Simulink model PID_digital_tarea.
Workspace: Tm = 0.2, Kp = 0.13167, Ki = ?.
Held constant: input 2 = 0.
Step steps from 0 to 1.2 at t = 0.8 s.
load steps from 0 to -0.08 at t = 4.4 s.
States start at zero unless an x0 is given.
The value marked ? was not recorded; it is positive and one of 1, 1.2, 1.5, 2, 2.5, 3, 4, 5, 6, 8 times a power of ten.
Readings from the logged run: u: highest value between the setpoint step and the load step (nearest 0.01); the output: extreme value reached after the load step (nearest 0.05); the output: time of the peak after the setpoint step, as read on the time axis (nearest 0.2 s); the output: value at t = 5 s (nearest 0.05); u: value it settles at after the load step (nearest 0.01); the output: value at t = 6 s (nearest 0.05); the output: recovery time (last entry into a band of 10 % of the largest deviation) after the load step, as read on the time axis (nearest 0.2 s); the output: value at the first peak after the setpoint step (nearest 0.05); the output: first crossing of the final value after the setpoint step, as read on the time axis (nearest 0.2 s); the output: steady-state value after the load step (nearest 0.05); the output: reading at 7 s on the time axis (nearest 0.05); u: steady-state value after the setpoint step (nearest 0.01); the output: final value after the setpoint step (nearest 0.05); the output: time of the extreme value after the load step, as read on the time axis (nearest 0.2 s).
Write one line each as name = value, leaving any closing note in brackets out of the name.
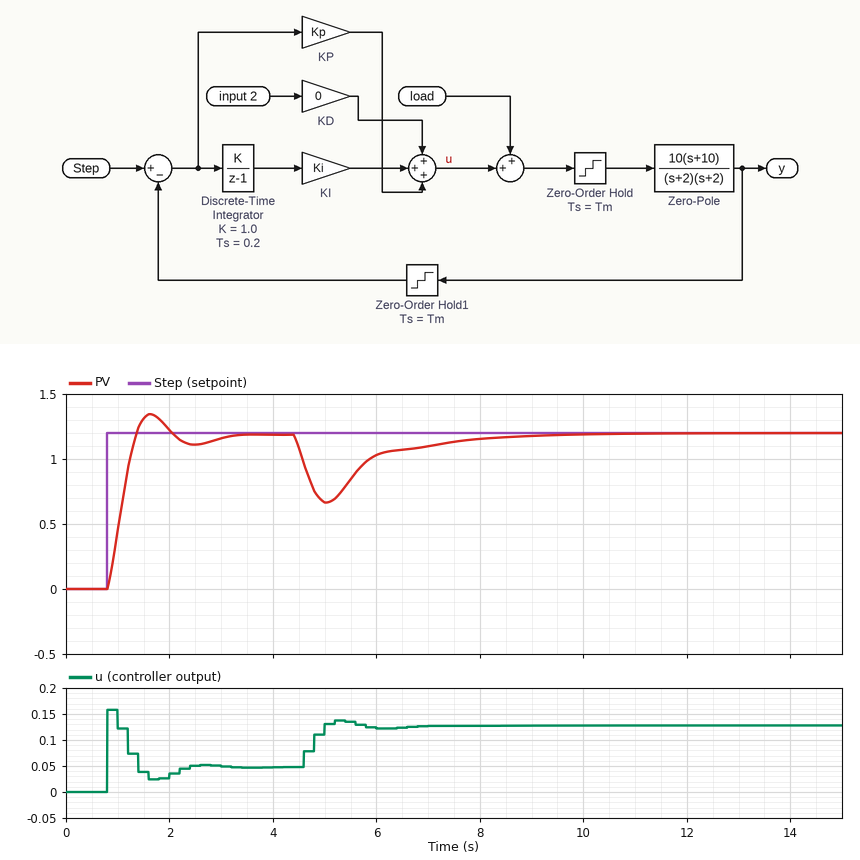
u: highest value between the setpoint step and the load step = 0.16
the output: extreme value reached after the load step = 0.65
the output: time of the peak after the setpoint step, as read on the time axis = 1.6 s
the output: value at t = 5 s = 0.65
u: value it settles at after the load step = 0.13
the output: value at t = 6 s = 1.05
the output: recovery time (last entry into a band of 10 % of the largest deviation) after the load step, as read on the time axis = 7.8 s
the output: value at the first peak after the setpoint step = 1.35
the output: first crossing of the final value after the setpoint step, as read on the time axis = 1.4 s
the output: steady-state value after the load step = 1.20
the output: reading at 7 s on the time axis = 1.10
u: steady-state value after the setpoint step = 0.05
the output: final value after the setpoint step = 1.20
the output: time of the extreme value after the load step, as read on the time axis = 5.0 s
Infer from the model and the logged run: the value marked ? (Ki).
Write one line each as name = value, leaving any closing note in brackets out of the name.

the value marked ? = 0.02
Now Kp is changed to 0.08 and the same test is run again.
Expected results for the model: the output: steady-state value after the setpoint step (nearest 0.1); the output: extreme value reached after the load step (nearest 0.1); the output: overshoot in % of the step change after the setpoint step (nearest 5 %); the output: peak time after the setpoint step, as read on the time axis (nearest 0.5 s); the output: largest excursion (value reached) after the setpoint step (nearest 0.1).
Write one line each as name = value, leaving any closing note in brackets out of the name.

the output: steady-state value after the setpoint step = 1.2
the output: extreme value reached after the load step = 0.5
the output: overshoot in % of the step change after the setpoint step = 15 %
the output: peak time after the setpoint step, as read on the time axis = 2.0 s
the output: largest excursion (value reached) after the setpoint step = 1.4
